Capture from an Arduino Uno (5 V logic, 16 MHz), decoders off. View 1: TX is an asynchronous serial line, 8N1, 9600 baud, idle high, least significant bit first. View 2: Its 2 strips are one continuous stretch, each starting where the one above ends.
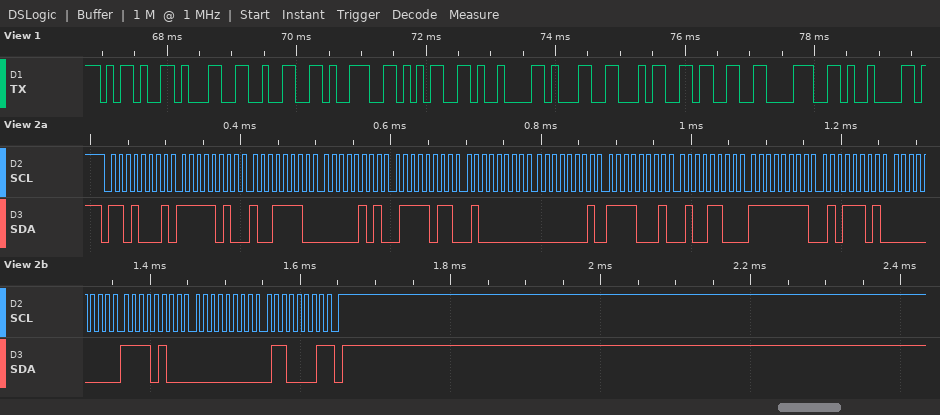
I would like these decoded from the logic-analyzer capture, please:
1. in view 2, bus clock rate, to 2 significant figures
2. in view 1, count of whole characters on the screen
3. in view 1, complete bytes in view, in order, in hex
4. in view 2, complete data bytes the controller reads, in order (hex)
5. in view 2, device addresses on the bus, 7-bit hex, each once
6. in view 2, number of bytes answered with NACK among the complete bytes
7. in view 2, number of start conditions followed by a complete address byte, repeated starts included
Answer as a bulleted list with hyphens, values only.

- 100 kHz
- 11
- 0x2D 0x31 0x32 0x39 0x35 0x09 0x31 0x34 0x33 0x38 0x09
- FA 9E 05 7B 40 01 F1 4C FF 5D 00 F4 00 61
- 0x68
- 1
- 1
